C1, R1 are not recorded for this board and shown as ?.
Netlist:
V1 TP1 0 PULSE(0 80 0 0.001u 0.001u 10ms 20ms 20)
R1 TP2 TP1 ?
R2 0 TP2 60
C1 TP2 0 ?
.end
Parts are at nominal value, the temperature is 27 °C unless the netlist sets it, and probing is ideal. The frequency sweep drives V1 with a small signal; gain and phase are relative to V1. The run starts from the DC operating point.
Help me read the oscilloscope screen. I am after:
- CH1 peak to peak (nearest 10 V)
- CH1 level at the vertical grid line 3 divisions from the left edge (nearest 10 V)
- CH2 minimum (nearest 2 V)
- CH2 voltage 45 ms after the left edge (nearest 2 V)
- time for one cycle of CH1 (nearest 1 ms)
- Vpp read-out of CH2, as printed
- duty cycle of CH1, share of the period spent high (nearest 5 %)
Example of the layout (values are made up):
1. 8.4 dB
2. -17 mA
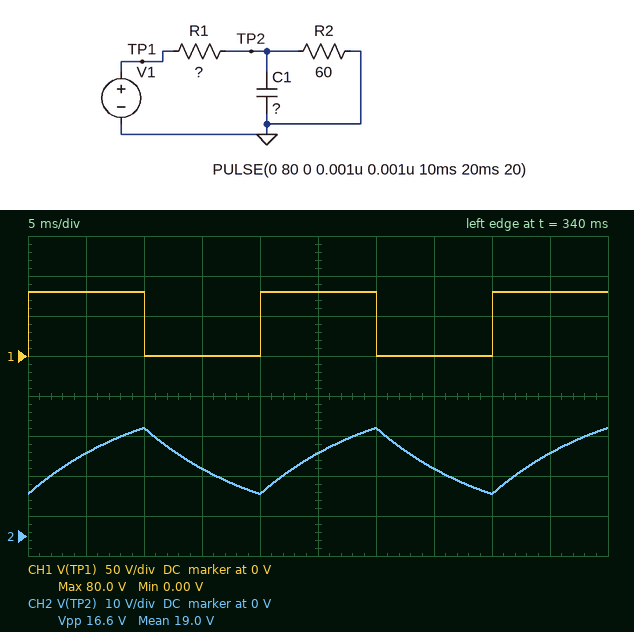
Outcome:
1. 80 V
2. 0 V
3. 10 V
4. 20 V
5. 20 ms
6. 16.6 V
7. 50 %
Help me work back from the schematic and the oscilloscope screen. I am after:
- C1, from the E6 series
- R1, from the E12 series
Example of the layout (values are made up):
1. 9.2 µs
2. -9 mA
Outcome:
1. 330 µF
2. 68 Ω
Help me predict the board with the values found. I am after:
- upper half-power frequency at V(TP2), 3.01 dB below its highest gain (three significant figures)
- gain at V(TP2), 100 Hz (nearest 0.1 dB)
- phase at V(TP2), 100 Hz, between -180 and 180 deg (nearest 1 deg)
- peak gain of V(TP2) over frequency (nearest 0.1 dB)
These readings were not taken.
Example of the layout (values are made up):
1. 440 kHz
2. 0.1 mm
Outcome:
1. 15.1 Hz
2. -23.1 dB
3. -81 deg
4. -6.6 dB
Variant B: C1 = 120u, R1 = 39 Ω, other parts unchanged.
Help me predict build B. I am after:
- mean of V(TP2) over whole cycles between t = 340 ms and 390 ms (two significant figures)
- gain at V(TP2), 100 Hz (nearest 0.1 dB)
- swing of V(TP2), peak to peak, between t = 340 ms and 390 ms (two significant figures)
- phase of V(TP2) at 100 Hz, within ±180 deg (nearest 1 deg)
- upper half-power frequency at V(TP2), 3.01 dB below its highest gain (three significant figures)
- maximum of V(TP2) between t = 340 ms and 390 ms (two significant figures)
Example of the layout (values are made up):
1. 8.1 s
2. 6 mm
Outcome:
1. 24 V
2. -10.6 dB
3. 46 V
4. -61 deg
5. 56.1 Hz
6. 47 V
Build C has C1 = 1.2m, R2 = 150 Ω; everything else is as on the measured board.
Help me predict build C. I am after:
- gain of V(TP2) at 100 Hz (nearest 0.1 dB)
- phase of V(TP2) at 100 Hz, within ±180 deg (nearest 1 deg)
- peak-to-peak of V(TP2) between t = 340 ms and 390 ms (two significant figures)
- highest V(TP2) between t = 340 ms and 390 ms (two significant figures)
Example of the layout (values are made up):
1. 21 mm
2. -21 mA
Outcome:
1. -34.2 dB
2. -88 deg
3. 4.9 V
4. 30 V
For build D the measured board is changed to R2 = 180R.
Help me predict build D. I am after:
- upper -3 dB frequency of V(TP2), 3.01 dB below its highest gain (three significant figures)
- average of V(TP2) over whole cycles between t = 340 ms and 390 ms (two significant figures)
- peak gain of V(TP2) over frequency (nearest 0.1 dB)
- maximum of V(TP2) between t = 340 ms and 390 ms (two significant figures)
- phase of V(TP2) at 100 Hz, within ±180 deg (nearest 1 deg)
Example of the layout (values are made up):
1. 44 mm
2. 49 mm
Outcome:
1. 9.77 Hz
2. 29 V
3. -2.8 dB
4. 38 V
5. -84 deg
